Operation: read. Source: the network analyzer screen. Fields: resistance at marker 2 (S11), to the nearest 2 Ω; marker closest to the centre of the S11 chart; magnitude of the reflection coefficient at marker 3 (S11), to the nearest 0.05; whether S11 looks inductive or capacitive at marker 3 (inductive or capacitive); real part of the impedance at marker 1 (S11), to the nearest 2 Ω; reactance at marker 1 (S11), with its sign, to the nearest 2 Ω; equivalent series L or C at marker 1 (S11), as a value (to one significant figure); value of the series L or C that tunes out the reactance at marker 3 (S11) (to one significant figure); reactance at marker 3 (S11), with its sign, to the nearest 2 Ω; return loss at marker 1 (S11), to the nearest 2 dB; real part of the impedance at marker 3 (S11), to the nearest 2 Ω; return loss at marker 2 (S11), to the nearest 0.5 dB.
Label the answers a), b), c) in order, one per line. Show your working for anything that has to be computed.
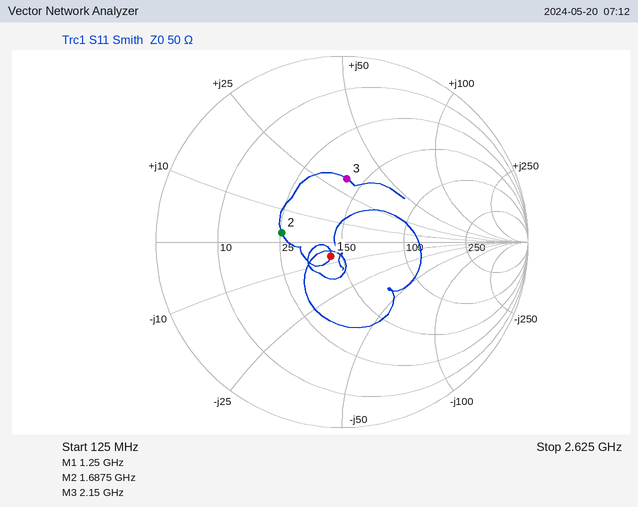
a) 26 Ω
b) marker 1
c) 0.35
d) inductive
e) 44 Ω
f) -6 Ω
g) C = 1/(2π × 1.25 GHz × 6 Ω) ≈ 21.2 pF, so 20 pF to one significant figure
h) C = 1/(2π × 2.15 GHz × 32 Ω) ≈ 2 pF
i) +32 Ω
j) 20 dB
k) 42 Ω
l) 9.5 dB
